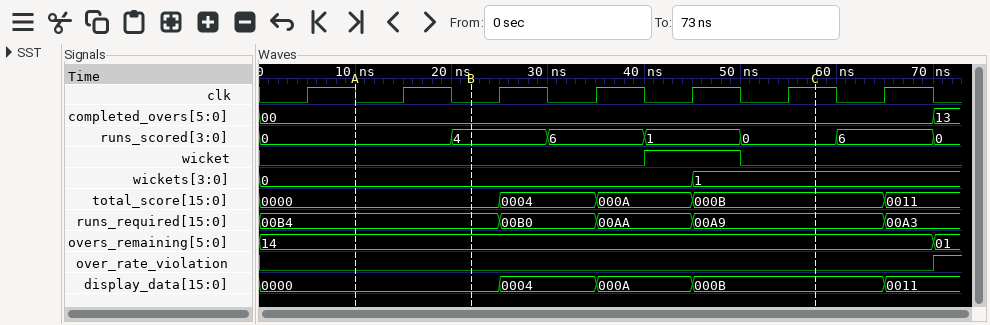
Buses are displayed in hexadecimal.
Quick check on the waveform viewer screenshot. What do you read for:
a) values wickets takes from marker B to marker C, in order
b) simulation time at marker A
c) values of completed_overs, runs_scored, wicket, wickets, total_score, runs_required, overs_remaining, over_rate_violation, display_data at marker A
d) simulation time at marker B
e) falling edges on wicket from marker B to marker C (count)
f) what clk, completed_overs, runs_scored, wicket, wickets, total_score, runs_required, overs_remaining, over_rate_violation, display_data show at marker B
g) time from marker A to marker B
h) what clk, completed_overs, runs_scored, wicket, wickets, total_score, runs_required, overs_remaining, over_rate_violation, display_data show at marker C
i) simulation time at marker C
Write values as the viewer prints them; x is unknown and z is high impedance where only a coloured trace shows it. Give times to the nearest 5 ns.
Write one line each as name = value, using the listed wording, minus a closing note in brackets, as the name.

values wickets takes from marker B to marker C, in order = 0, 1
simulation time at marker A = 10 ns
values of completed_overs, runs_scored, wicket, wickets, total_score, runs_required, overs_remaining, over_rate_violation, display_data at marker A = completed_overs=00, runs_scored=0, wicket=0, wickets=0, total_score=0000, runs_required=00B4, overs_remaining=14, over_rate_violation=0, display_data=0000
simulation time at marker B = 20 ns
falling edges on wicket from marker B to marker C = 1
what clk, completed_overs, runs_scored, wicket, wickets, total_score, runs_required, overs_remaining, over_rate_violation, display_data show at marker B = clk=0, completed_overs=00, runs_scored=4, wicket=0, wickets=0, total_score=0000, runs_required=00B4, overs_remaining=14, over_rate_violation=0, display_data=0000
time from marker A to marker B = 10 ns
what clk, completed_overs, runs_scored, wicket, wickets, total_score, runs_required, overs_remaining, over_rate_violation, display_data show at marker C = clk=1, completed_overs=00, runs_scored=0, wicket=0, wickets=1, total_score=000B, runs_required=00A9, overs_remaining=14, over_rate_violation=0, display_data=000B
simulation time at marker C = 60 ns
